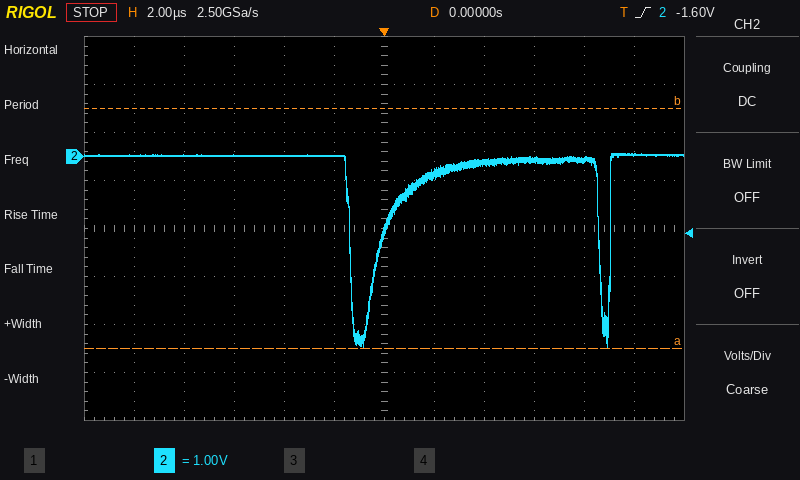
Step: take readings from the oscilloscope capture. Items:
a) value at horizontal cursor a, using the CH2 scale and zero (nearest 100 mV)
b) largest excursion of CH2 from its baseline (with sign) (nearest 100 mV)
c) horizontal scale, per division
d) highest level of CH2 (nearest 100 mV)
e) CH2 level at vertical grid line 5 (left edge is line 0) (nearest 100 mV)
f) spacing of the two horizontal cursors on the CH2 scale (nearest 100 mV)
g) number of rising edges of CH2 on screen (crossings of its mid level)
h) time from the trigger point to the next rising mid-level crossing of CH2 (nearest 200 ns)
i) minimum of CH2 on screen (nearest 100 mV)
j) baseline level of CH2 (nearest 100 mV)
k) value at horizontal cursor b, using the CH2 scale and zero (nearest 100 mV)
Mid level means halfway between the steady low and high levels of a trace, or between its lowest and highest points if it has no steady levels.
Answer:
-4.0 V
-4.0 V
2 µs
100 mV
0.0 V
5.0 V
2
9.0 µs
-4.0 V
0.0 V
1.0 V
